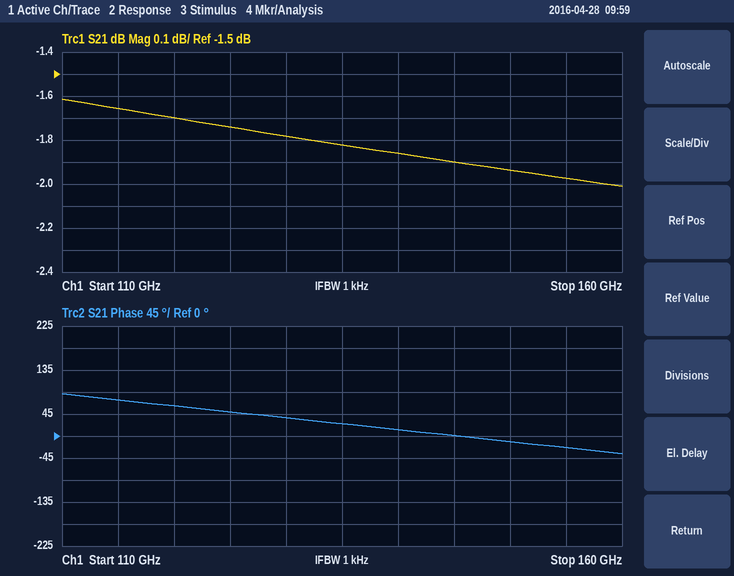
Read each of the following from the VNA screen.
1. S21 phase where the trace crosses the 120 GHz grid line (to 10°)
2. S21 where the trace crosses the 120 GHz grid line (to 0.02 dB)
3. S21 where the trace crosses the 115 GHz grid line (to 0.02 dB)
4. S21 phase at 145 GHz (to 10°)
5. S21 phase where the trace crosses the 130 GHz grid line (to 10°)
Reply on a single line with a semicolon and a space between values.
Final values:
60°; -1.70 dB; -1.66 dB; 0°; 40°
